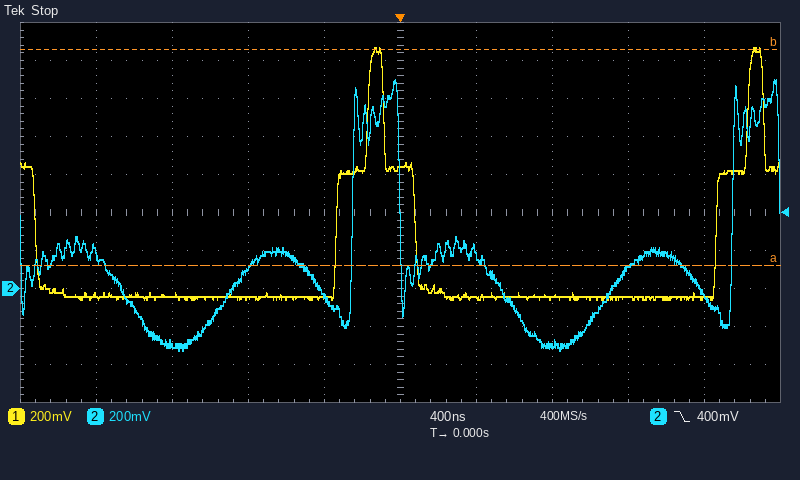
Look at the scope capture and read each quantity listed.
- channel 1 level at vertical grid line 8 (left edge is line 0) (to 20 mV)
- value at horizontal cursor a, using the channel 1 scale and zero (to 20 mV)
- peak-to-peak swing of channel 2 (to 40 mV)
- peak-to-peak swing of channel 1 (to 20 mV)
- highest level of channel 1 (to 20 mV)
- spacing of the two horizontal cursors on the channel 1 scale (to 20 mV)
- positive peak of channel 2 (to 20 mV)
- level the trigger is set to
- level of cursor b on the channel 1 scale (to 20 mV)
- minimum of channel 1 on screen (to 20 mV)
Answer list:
-40 mV
120 mV
1.44 V
1.32 V
1.26 V
1.14 V
1.10 V
400 mV
1.26 V
-60 mV
